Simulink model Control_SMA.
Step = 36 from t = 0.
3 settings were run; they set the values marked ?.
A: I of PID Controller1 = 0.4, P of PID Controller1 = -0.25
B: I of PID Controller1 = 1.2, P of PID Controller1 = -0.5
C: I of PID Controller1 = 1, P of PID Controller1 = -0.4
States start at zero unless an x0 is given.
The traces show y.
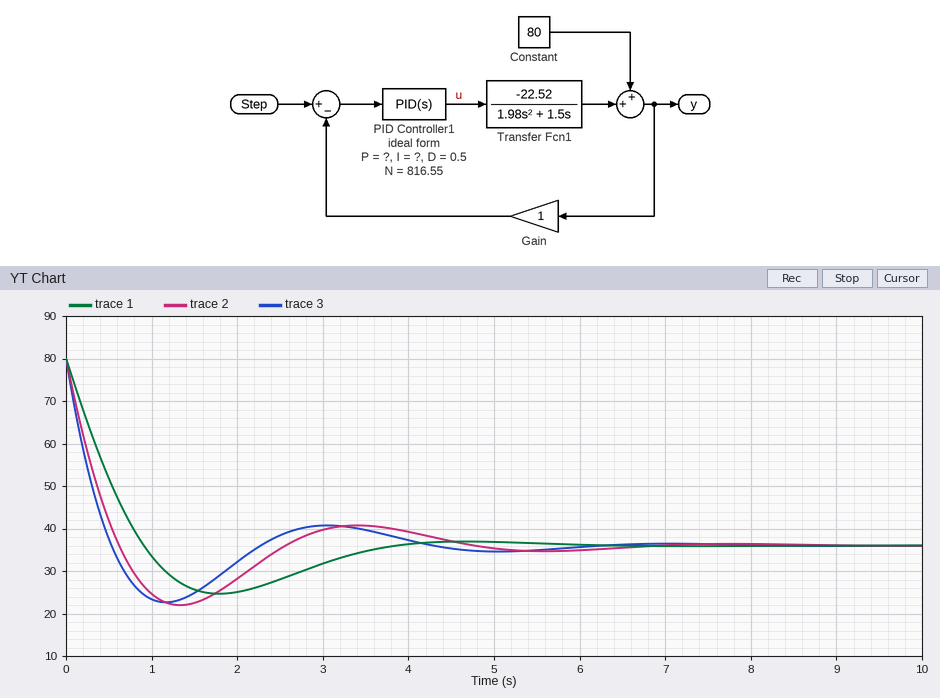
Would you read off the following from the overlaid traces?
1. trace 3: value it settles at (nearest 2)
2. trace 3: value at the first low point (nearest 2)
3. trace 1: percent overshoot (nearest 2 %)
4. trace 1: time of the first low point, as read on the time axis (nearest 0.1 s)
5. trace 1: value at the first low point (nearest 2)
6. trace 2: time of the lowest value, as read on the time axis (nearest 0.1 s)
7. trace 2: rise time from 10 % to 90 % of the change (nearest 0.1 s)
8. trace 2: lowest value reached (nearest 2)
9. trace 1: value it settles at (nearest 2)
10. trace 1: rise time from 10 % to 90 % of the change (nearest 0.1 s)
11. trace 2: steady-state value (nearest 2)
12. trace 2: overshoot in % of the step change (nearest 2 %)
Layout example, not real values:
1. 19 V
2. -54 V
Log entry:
1. 36
2. 22
3. 26 %
4. 1.8 s
5. 24
6. 1.3 s
7. 0.5 s
8. 22
9. 36
10. 0.7 s
11. 36
12. 32 %
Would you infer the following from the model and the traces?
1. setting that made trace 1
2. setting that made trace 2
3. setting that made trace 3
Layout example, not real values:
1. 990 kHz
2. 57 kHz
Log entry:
1. A
2. C
3. B
